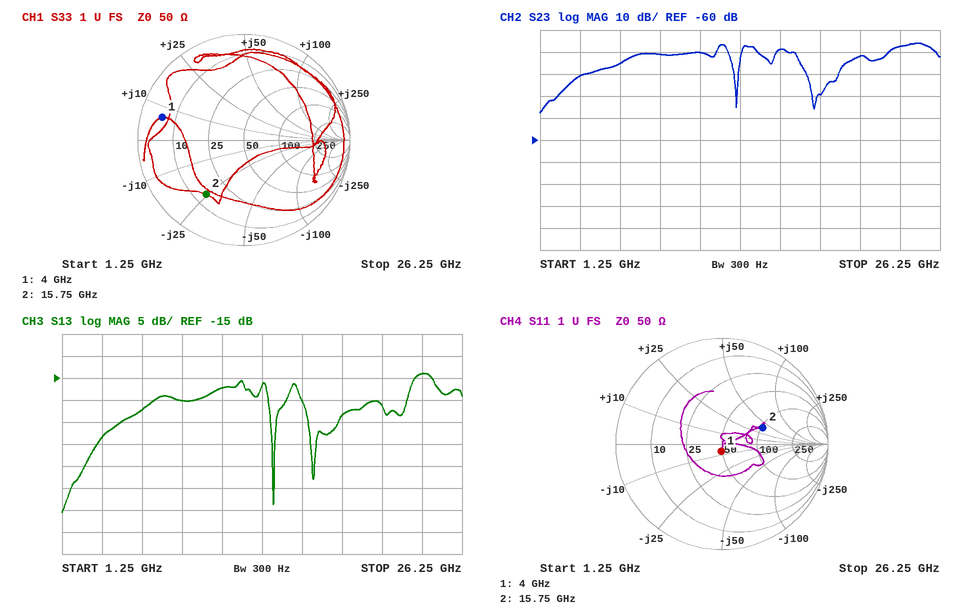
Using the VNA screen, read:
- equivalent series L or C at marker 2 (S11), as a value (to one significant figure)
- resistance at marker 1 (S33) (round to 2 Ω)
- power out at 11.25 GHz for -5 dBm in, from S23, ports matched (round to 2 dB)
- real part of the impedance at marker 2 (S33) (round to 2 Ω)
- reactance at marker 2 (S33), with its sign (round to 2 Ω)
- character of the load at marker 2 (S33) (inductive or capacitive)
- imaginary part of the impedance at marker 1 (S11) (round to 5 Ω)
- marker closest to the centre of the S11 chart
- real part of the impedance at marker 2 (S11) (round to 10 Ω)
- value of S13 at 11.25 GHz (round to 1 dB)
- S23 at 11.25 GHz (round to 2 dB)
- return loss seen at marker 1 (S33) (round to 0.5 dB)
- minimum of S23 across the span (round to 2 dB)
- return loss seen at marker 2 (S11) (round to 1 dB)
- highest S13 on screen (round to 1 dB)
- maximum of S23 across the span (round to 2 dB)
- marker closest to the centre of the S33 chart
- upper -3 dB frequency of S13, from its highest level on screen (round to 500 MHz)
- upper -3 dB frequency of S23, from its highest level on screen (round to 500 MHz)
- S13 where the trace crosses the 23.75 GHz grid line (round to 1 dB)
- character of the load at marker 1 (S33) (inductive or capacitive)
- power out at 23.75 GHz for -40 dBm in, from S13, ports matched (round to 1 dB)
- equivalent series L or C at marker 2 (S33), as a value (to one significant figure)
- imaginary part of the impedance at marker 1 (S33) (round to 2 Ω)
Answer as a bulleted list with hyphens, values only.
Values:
- 400 pH
- 6 Ω
- -26 dBm
- 14 Ω
- -24 Ω
- capacitive
- -5 Ω
- marker 1
- 100 Ω
- -17 dB
- -20 dB
- 2.0 dB
- -48 dB
- 8 dB
- -14 dB
- -16 dB
- marker 2
- 24.5 GHz
- 26.0 GHz
- -14 dB
- inductive
- -54 dBm
- 400 fF
- +6 Ω
